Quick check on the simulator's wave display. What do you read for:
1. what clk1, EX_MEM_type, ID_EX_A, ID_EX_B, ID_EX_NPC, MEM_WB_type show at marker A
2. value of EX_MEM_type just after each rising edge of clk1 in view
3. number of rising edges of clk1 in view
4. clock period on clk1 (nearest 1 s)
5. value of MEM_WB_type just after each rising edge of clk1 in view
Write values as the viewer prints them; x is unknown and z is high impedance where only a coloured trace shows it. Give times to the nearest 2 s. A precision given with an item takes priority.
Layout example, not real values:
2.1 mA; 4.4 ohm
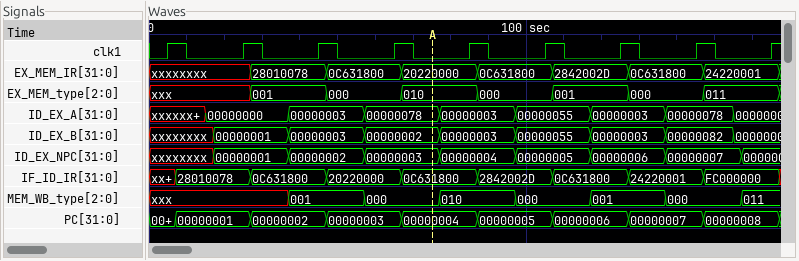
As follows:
clk1=0, EX_MEM_type=010, ID_EX_A=00000078, ID_EX_B=00000002, ID_EX_NPC=00000003, MEM_WB_type=000; xxx, xxx, 001, 000, 010, 000, 001, 000, 011; 9; 20 s; xxx, xxx, 001, 000, 010, 000, 001, 000, 011
